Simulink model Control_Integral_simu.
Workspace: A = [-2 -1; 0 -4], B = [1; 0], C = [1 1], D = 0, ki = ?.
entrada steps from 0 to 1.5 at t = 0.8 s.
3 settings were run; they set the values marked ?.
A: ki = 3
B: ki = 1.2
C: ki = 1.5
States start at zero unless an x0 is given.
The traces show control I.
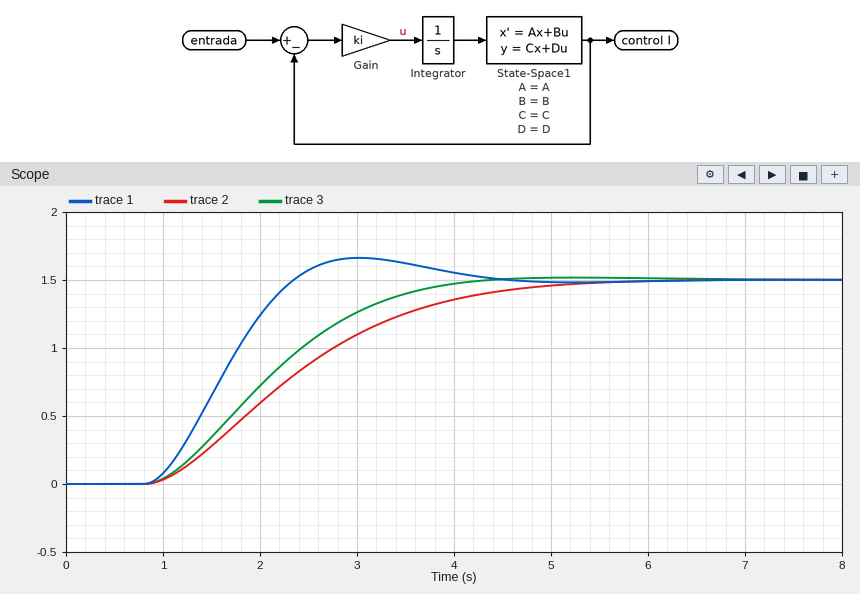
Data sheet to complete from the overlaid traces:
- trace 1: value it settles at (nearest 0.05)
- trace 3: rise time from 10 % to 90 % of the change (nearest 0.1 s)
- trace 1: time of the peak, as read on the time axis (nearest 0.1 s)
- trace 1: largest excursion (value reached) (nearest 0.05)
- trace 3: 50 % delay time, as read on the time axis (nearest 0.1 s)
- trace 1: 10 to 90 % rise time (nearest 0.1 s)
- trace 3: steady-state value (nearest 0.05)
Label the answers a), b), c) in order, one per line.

a) 1.50
b) 2.1 s
c) 3.0 s
d) 1.65
e) 2.0 s
f) 1.0 s
g) 1.50
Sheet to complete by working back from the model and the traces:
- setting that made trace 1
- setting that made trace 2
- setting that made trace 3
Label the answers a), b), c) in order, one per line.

a) A
b) B
c) C
